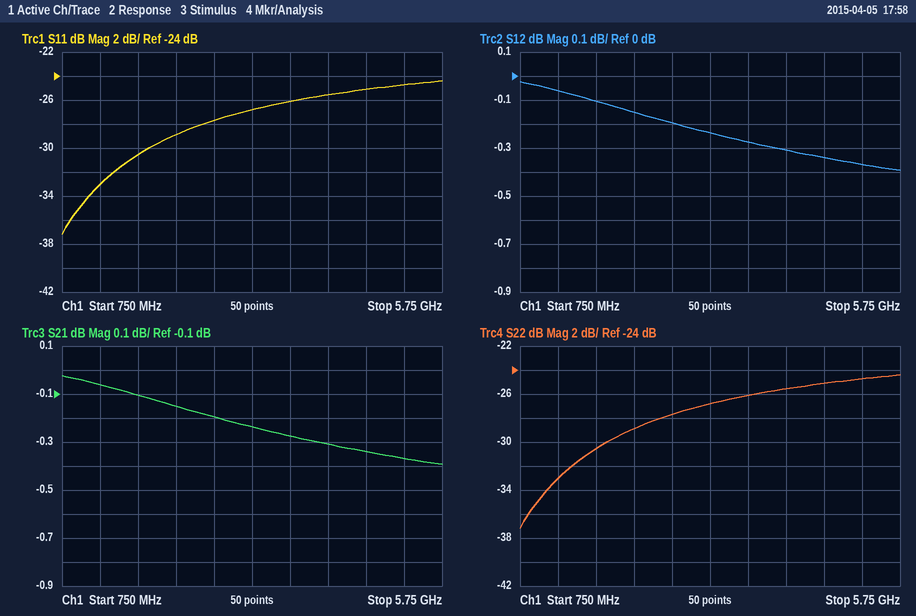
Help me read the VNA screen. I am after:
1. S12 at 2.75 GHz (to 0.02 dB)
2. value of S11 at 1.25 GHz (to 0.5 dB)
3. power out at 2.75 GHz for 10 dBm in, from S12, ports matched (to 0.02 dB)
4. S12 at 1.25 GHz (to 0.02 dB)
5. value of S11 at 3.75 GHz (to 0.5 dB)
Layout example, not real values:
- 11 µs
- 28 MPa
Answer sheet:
- -0.20 dB
- -33.0 dB
- 9.80 dBm
- -0.06 dB
- -26.0 dB
